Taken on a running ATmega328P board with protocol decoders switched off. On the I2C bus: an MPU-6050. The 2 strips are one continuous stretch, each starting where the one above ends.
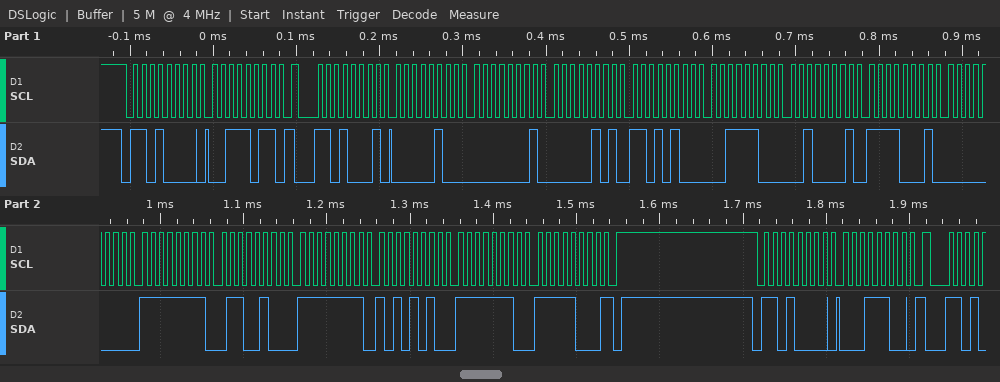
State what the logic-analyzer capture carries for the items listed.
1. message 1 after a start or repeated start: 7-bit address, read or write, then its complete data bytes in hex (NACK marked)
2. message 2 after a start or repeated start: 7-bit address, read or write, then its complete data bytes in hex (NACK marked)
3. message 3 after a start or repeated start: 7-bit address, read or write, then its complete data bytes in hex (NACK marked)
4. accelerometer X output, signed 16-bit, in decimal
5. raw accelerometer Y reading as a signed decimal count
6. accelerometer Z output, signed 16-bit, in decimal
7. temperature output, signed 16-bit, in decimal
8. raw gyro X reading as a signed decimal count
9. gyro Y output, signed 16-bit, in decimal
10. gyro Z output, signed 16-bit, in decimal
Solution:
0x68 write: 3B
0x68 read: 04 01 05 D4 3C 21 F1 00 FF 64 FF AA FE F8 NACK
0x68 write: 1C
1025
1492
15393
-3840
-156
-86
-264
